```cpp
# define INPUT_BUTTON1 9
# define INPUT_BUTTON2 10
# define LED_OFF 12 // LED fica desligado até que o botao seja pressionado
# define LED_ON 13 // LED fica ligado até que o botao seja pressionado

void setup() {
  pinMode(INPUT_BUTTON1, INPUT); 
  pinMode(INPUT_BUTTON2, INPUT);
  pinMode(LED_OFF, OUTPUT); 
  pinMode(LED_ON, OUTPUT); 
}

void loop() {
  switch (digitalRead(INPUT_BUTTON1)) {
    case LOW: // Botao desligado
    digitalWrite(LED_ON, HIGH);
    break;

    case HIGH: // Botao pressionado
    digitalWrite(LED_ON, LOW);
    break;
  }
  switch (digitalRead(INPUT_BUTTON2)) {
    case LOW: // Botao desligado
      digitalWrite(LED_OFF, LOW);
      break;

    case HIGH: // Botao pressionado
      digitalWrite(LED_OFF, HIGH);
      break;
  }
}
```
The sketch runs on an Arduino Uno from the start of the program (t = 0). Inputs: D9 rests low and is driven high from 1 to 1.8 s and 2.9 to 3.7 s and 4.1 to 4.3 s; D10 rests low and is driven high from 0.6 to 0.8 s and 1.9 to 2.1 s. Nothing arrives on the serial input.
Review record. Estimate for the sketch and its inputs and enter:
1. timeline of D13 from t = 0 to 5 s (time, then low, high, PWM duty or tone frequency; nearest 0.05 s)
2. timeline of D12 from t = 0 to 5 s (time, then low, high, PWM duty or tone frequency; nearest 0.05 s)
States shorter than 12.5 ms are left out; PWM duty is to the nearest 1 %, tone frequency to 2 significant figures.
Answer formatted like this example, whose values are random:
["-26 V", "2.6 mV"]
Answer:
["0 s high; 1 s low; 1.8 s high; 2.9 s low; 3.7 s high; 4.1 s low; 4.3 s high", "0 s low; 0.6 s high; 0.8 s low; 1.9 s high; 2.1 s low"]
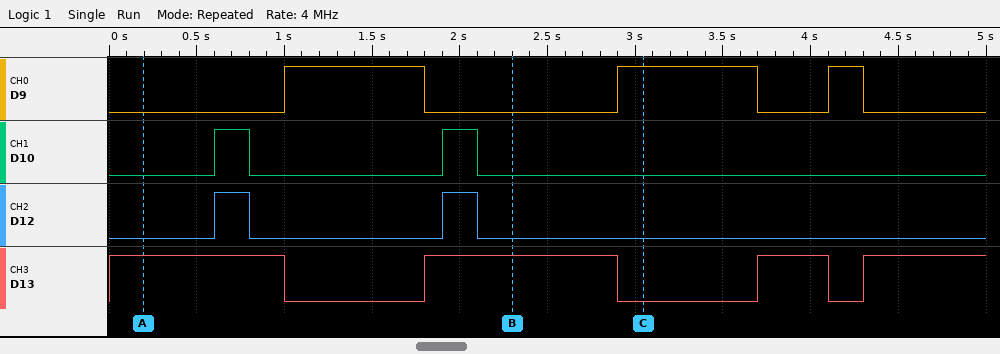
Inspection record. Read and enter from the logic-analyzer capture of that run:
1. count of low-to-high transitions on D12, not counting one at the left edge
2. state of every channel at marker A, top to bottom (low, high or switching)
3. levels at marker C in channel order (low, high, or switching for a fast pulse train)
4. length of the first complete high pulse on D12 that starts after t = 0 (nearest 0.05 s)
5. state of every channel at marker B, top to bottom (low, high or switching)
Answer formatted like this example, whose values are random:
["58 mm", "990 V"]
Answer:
["2", "D9 low, D10 low, D12 low, D13 high", "D9 high, D10 low, D12 low, D13 low", "0.20 s", "D9 low, D10 low, D12 low, D13 high"]
